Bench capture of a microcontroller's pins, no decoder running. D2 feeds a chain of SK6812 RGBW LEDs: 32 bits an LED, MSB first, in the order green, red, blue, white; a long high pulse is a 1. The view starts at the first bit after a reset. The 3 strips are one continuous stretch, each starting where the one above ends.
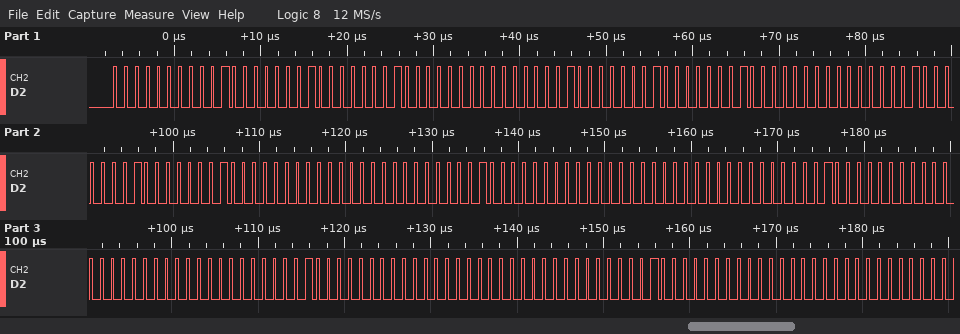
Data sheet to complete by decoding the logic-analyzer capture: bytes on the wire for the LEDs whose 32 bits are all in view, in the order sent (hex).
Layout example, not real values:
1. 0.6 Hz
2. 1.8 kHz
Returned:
1. 00 20 20 20 00 20 20 20 00 20 20 20 00 00 20 00 00 00 20 00 00 00 20 00 00 00 20 00
